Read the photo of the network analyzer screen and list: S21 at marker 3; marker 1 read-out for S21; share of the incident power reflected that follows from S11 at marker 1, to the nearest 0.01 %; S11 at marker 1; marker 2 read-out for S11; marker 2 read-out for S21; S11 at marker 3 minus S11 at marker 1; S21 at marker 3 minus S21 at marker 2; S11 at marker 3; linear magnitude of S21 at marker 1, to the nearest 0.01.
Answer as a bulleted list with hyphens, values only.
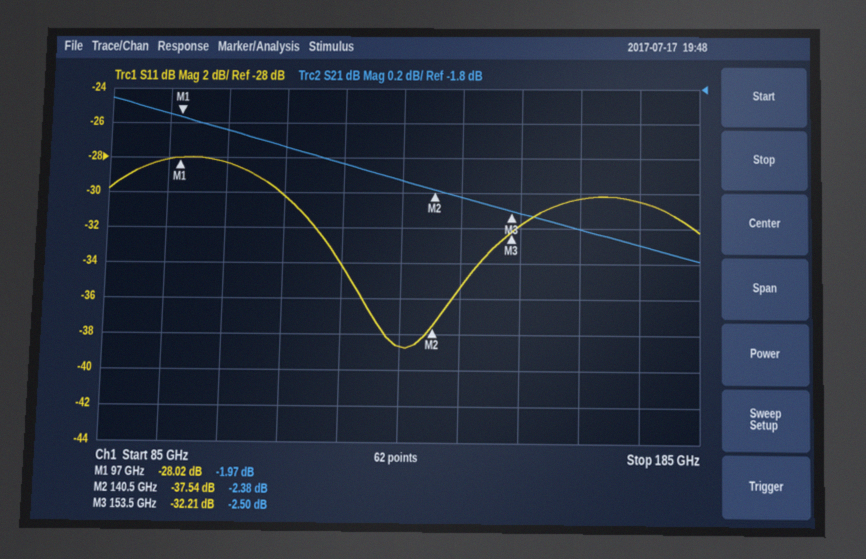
- -2.50 dB
- -1.97 dB
- 0.16 %
- -28.02 dB
- -37.54 dB
- -2.38 dB
- -4.19 dB
- -0.12 dB
- -32.21 dB
- 0.80
